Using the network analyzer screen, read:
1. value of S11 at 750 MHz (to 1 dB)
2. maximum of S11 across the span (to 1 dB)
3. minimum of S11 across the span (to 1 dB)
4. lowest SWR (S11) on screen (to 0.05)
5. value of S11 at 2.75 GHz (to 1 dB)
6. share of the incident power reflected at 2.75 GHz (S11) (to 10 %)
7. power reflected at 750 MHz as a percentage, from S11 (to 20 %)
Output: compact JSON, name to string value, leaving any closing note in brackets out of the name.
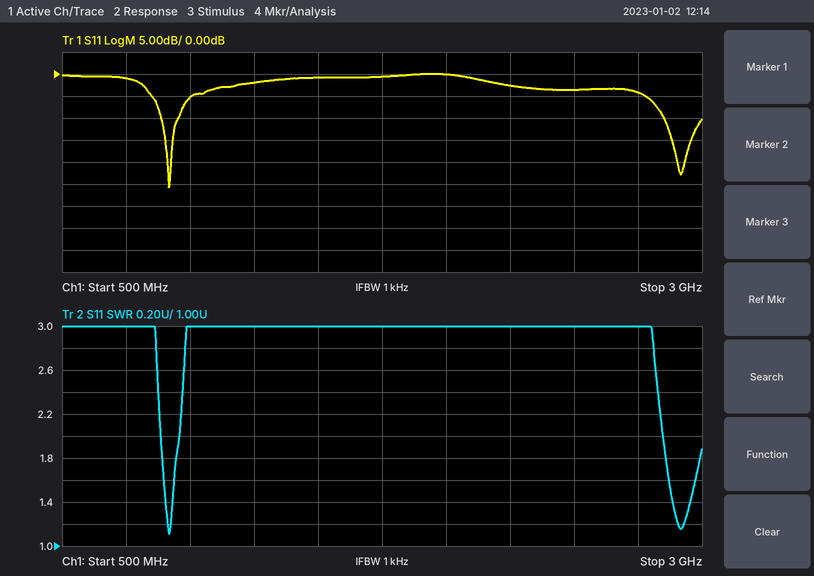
{"value of S11 at 750 MHz": "-1 dB", "maximum of S11 across the span": "0 dB", "minimum of S11 across the span": "-26 dB", "lowest SWR (S11) on screen": "1.10", "value of S11 at 2.75 GHz": "-4 dB", "share of the incident power reflected at 2.75 GHz (S11)": "40 %", "power reflected at 750 MHz as a percentage, from S11": "80 %"}
